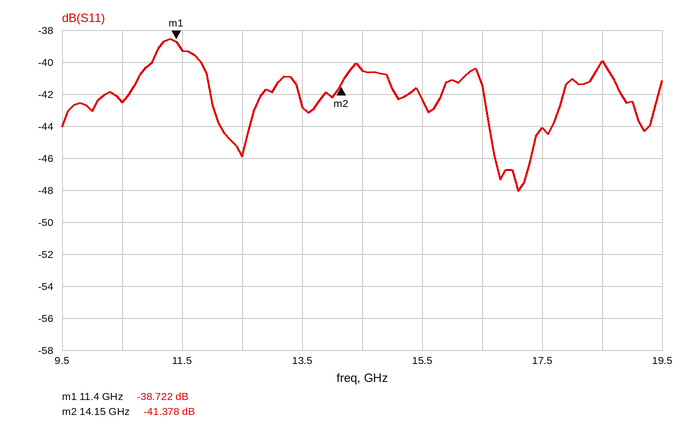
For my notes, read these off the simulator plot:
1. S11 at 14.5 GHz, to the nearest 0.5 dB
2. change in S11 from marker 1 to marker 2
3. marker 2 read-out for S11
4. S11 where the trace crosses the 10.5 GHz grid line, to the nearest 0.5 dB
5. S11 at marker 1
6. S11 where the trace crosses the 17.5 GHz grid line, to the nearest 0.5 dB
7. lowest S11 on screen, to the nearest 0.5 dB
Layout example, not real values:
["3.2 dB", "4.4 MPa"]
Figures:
["-40.5 dB", "-2.656 dB", "-41.378 dB", "-42.5 dB", "-38.722 dB", "-44.0 dB", "-48.0 dB"]
